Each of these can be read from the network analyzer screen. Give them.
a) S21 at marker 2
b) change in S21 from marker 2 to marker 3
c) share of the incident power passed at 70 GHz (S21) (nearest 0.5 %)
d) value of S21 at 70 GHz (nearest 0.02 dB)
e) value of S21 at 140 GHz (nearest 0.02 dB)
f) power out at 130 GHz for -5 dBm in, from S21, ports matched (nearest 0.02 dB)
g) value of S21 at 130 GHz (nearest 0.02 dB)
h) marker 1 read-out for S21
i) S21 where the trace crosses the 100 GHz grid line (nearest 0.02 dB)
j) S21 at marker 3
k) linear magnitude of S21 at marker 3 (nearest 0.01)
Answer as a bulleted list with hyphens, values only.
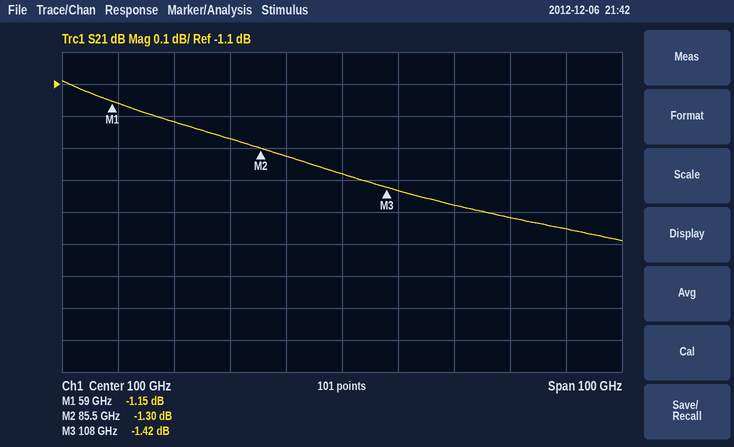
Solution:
- -1.30 dB
- -0.12 dB
- 75.5 %
- -1.22 dB
- -1.56 dB
- -6.52 dBm
- -1.52 dB
- -1.15 dB
- -1.38 dB
- -1.42 dB
- 0.85
